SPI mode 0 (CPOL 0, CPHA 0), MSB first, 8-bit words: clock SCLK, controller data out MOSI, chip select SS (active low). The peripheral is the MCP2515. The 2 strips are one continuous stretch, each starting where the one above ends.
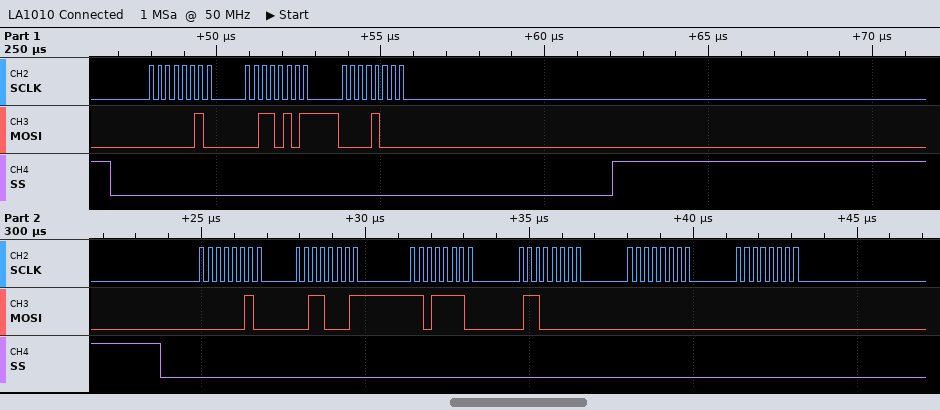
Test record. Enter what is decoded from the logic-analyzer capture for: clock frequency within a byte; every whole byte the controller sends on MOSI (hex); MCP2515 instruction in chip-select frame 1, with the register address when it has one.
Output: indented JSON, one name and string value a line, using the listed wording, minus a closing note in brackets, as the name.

{
  "clock frequency within a byte": "4 MHz",
  "every whole byte the controller sends on MOSI": "02 35 08 02 31 DE 60 00 00",
  "MCP2515 instruction in chip-select frame 1, with the register address when it has one": "WRITE 0x35"
}
